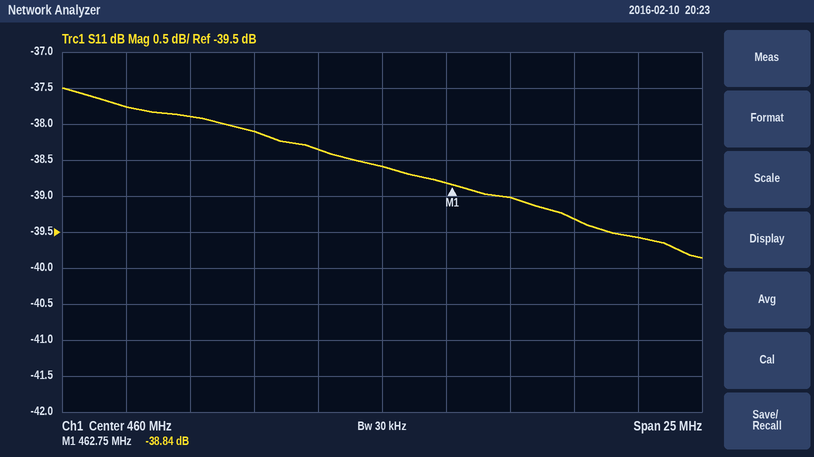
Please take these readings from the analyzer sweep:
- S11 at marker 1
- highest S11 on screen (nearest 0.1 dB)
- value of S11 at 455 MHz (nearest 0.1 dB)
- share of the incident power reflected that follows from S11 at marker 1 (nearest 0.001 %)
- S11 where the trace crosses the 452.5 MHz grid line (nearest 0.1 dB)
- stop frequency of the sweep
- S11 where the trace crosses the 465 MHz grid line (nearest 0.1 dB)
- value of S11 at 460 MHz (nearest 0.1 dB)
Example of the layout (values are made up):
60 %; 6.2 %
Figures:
-38.84 dB; -37.5 dB; -38.1 dB; 0.013 %; -37.9 dB; 472.5 MHz; -39.0 dB; -38.6 dB
